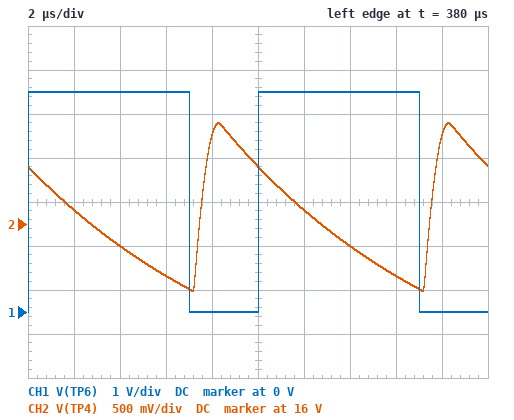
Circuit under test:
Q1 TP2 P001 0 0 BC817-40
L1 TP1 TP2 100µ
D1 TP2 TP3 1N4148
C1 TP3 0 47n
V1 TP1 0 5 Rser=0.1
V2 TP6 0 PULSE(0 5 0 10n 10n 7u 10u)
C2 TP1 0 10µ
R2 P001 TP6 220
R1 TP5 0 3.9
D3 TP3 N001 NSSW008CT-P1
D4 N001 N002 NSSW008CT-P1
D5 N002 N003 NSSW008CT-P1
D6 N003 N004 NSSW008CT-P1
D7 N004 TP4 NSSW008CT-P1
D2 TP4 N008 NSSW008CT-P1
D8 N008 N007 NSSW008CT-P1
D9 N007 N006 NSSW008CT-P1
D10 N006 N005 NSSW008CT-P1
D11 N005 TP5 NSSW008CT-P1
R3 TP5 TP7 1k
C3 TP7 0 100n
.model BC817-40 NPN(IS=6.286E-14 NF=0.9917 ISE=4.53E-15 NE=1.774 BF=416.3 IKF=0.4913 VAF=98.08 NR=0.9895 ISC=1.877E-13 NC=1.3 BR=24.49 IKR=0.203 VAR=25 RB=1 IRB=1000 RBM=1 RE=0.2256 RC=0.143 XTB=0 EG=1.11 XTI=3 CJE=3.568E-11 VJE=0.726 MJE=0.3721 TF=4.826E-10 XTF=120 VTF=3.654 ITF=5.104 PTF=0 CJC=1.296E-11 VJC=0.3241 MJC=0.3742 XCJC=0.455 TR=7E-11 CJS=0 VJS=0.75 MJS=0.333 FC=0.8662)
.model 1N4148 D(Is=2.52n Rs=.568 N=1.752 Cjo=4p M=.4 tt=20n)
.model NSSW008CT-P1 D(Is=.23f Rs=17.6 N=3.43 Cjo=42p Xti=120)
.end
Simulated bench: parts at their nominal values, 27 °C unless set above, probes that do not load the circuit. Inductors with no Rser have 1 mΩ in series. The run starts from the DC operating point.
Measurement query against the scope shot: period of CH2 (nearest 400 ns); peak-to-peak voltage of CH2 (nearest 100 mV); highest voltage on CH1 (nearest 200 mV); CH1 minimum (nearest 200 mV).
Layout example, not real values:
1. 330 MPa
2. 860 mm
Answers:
1. 10.0 µs
2. 1.9 V
3. 5.0 V
4. 0 V
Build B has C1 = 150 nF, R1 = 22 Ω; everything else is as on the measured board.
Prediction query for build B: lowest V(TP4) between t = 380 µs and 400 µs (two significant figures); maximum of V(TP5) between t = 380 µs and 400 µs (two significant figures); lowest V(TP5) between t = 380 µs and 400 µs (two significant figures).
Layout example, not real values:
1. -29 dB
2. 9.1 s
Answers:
1. 16 V
2. 500 mV
3. 390 mV
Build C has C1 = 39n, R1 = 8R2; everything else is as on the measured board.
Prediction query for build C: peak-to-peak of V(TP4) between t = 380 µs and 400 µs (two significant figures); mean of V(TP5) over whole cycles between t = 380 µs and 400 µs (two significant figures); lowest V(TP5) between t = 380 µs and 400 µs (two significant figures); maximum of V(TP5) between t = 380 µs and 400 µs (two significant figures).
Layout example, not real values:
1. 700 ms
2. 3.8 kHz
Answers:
1. 2.3 V
2. 170 mV
3. 98 mV
4. 260 mV
